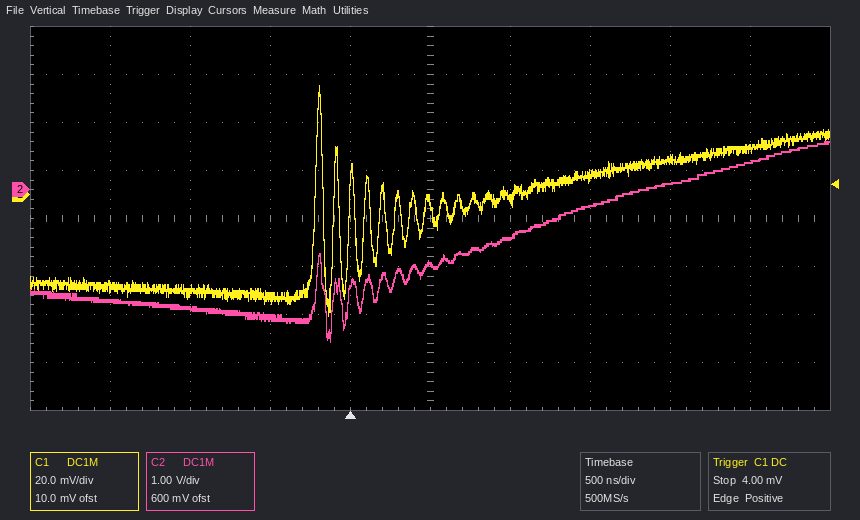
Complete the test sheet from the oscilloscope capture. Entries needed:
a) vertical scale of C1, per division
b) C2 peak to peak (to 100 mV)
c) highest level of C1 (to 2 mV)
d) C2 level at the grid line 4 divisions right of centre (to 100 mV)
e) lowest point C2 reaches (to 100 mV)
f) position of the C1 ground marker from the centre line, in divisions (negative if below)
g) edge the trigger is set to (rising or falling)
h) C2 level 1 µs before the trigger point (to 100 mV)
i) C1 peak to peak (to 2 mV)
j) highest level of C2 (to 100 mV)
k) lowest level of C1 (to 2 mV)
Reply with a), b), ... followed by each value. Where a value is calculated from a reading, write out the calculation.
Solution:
a) 20 mV
b) 1.0 V − (-3.2 V) = 4.2 V
c) 46 mV
d) 600 mV
e) -3.2 V
f) +0.5 div
g) rising
h) -2.5 V
i) 46 mV − (-50 mV) = 96 mV
j) 1.0 V
k) -50 mV
